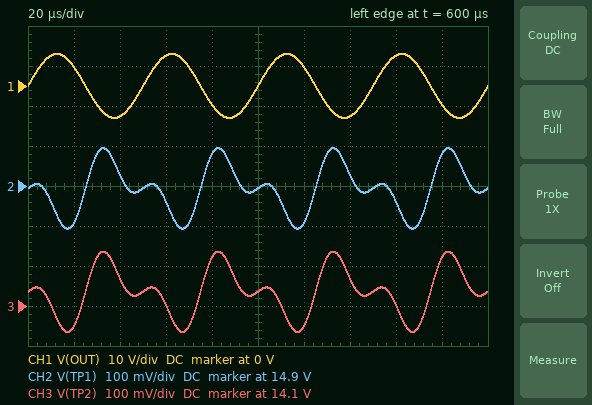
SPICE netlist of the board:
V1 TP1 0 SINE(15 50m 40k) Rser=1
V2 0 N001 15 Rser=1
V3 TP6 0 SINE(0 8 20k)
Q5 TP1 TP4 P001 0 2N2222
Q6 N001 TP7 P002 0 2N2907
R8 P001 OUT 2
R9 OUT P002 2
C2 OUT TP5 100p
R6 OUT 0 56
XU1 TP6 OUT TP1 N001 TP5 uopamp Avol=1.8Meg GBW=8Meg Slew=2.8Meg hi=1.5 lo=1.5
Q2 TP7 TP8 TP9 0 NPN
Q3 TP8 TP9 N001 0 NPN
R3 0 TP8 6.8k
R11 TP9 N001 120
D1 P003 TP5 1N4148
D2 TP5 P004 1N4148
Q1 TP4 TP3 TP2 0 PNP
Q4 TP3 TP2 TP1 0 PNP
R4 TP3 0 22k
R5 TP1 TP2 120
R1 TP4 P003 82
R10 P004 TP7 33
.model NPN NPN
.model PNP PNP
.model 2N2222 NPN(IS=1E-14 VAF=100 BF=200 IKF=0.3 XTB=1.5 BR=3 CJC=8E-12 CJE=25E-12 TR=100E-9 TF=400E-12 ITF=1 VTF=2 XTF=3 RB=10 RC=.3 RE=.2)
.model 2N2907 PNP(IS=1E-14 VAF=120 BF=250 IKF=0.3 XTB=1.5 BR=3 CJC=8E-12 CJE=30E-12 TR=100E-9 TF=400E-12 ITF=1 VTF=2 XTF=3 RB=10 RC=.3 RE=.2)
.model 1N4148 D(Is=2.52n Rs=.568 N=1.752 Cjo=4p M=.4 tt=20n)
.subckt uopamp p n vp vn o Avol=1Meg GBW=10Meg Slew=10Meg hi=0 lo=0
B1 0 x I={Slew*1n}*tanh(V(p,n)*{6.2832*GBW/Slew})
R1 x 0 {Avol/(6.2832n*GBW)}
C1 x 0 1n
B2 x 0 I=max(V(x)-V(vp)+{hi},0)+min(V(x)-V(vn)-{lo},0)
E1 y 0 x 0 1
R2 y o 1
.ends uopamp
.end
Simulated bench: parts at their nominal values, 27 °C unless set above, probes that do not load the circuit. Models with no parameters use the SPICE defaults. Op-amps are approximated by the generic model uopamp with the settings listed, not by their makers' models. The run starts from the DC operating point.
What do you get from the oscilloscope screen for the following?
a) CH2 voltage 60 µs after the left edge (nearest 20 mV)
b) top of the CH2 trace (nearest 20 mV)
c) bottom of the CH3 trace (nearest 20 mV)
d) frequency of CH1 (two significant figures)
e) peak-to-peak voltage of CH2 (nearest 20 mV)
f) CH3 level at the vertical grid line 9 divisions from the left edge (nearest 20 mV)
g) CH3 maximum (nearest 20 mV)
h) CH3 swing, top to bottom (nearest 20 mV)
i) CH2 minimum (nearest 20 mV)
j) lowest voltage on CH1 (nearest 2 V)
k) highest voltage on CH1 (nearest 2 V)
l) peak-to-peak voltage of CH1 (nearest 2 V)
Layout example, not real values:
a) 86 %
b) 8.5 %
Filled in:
a) 14.86 V
b) 15.00 V
c) 14.04 V
d) 20 kHz
e) 200 mV
f) 14.22 V
g) 14.24 V
h) 200 mV
i) 14.80 V
j) -8 V
k) 8 V
l) 16 V
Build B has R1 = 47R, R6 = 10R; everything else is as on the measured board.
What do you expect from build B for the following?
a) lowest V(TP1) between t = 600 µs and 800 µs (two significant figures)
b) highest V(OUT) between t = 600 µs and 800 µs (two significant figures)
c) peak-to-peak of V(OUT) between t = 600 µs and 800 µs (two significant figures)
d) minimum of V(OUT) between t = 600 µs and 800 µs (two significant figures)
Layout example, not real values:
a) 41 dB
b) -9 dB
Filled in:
a) 14 V
b) 5.2 V
c) 11 V
d) -6.0 V
